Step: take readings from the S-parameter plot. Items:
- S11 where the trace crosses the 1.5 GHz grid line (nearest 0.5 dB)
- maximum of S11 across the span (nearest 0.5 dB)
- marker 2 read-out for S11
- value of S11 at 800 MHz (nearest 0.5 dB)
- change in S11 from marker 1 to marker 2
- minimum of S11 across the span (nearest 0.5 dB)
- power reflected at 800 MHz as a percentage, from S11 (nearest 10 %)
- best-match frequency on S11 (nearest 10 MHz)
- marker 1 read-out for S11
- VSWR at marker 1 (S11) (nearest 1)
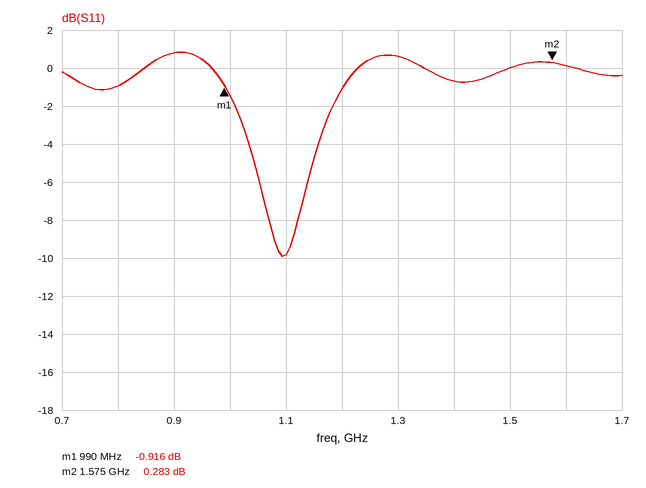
0.0 dB
1.0 dB
0.283 dB
-1.0 dB
1.199 dB
-10.0 dB
80 %
1.09 GHz
-0.916 dB
19
